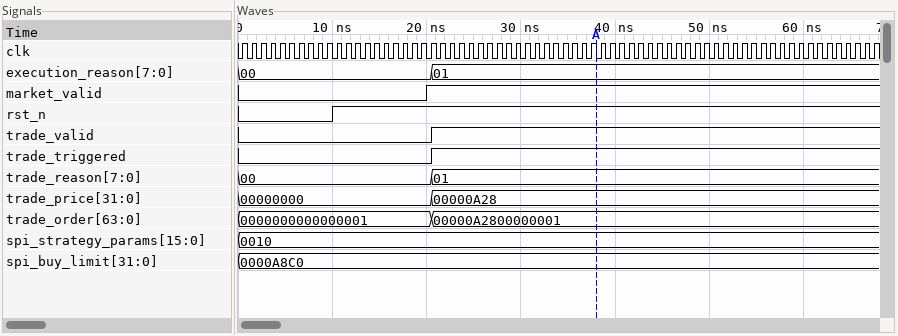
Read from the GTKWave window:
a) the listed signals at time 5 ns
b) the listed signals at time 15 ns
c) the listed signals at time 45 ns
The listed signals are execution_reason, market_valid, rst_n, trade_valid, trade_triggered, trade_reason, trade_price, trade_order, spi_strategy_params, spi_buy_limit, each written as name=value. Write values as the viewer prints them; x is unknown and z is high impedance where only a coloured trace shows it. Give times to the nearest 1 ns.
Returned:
execution_reason=00, market_valid=0, rst_n=0, trade_valid=0, trade_triggered=0, trade_reason=00, trade_price=00000000, trade_order=0000000000000001, spi_strategy_params=0010, spi_buy_limit=0000A8C0
execution_reason=00, market_valid=0, rst_n=1, trade_valid=0, trade_triggered=0, trade_reason=00, trade_price=00000000, trade_order=0000000000000001, spi_strategy_params=0010, spi_buy_limit=0000A8C0
execution_reason=01, market_valid=1, rst_n=1, trade_valid=1, trade_triggered=1, trade_reason=01, trade_price=00000A28, trade_order=00000A2800000001, spi_strategy_params=0010, spi_buy_limit=0000A8C0
